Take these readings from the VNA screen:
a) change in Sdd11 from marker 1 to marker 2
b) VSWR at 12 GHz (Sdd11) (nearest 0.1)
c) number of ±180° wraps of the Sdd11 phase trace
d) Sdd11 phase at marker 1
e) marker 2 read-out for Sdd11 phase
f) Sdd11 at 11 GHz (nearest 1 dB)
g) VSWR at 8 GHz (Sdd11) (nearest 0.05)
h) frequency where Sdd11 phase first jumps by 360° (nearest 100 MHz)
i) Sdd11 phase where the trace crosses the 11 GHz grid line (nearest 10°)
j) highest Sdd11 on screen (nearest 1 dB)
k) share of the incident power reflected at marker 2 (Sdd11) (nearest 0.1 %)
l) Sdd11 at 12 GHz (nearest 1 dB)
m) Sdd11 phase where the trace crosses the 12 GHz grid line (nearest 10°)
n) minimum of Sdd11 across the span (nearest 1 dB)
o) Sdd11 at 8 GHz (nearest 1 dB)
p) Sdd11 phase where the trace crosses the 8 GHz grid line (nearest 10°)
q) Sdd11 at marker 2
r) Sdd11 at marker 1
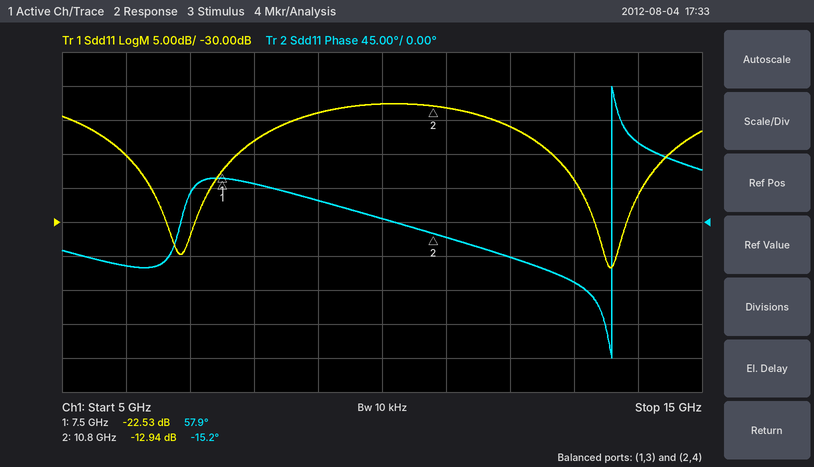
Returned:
9.59 dB
1.4
1
57.9°
-15.2°
-13 dB
1.30
13.6 GHz
-20°
-13 dB
5.1 %
-16 dB
-50°
-37 dB
-18 dB
50°
-12.94 dB
-22.53 dB
